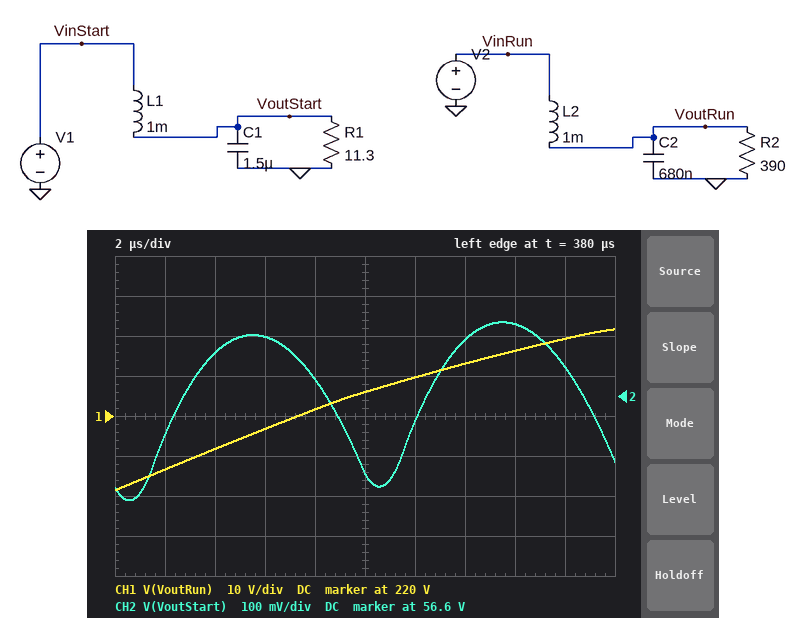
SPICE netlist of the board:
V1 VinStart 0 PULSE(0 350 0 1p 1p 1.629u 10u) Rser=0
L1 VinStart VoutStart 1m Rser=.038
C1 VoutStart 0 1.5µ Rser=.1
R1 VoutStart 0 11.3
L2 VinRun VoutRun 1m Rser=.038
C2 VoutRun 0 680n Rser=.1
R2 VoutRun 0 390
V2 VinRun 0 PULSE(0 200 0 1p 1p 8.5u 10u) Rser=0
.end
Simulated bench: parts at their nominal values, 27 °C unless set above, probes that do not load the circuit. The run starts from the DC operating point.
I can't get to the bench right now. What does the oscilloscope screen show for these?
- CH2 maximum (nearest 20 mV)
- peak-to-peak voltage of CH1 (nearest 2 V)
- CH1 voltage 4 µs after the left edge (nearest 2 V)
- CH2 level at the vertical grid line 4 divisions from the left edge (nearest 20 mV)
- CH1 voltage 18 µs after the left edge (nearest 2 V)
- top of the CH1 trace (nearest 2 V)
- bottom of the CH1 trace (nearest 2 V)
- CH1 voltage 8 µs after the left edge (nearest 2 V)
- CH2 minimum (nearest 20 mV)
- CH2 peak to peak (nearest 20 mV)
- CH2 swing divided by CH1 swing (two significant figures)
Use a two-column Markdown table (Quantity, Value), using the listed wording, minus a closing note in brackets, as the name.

| Quantity | Value |
|---|---|
| CH2 maximum | 56.78 V |
| peak-to-peak voltage of CH1 | 40 V |
| CH1 voltage 4 µs after the left edge | 212 V |
| CH2 level at the vertical grid line 4 divisions from the left edge | 56.64 V |
| CH1 voltage 18 µs after the left edge | 240 V |
| top of the CH1 trace | 242 V |
| bottom of the CH1 trace | 202 V |
| CH1 voltage 8 µs after the left edge | 222 V |
| CH2 minimum | 56.34 V |
| CH2 peak to peak | 440 mV |
| CH2 swing divided by CH1 swing | 0.011 |
